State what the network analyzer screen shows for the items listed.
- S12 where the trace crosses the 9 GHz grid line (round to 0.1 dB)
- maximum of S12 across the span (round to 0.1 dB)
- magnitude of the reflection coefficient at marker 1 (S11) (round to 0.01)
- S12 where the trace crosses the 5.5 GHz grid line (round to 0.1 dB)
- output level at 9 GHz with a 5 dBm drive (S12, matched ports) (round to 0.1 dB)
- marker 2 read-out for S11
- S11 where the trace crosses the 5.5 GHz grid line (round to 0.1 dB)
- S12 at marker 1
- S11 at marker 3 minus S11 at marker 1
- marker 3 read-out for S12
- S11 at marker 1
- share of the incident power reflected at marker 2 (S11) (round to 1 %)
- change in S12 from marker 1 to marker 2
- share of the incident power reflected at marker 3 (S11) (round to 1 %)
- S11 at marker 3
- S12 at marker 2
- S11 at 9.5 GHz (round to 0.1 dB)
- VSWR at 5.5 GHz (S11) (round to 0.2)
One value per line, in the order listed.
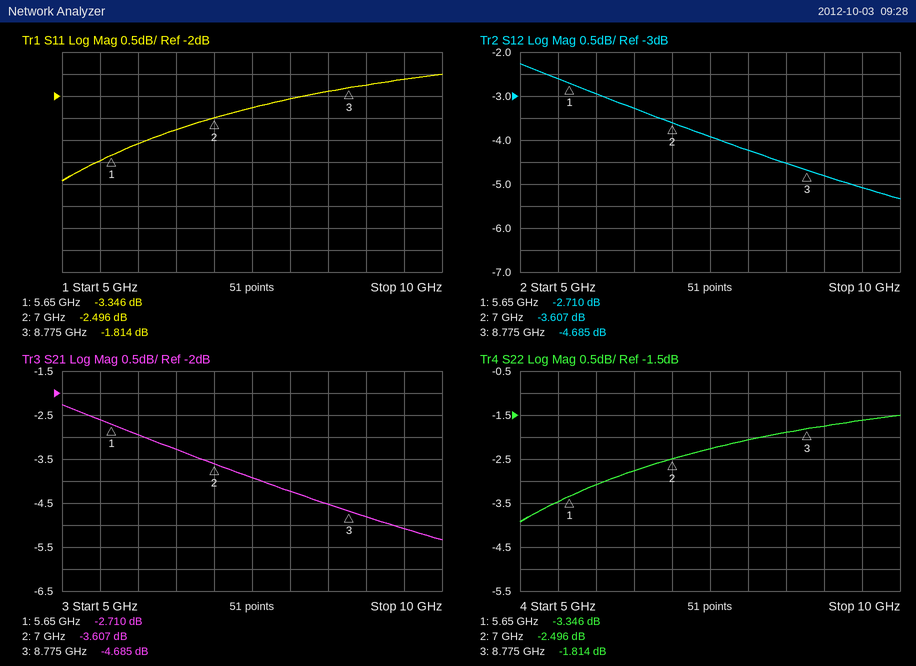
-4.8 dB
-2.3 dB
0.68
-2.6 dB
0.2 dBm
-2.496 dB
-3.5 dB
-2.710 dB
1.532 dB
-4.685 dB
-3.346 dB
56 %
-0.897 dB
66 %
-1.814 dB
-3.607 dB
-1.6 dB
5.0
